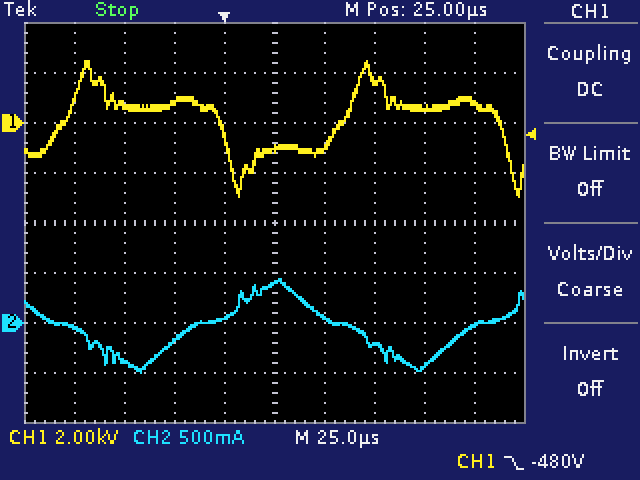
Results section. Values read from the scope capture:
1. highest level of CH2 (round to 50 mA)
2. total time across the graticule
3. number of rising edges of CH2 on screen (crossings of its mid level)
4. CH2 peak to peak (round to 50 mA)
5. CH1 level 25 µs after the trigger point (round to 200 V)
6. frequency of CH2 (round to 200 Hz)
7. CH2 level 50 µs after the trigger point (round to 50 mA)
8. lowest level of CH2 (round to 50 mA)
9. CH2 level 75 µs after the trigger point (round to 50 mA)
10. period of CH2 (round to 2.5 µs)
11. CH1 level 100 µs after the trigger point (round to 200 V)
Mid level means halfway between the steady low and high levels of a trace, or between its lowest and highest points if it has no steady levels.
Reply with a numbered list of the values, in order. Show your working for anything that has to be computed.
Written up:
1. 450 mA
2. 250 µs
3. 2
4. 450 mA − (-500 mA) = 950 mA
5. -1.0 kV
6. 1 / 140.0 µs ≈ 7.14 kHz, so 7.2 kHz to the nearest 200 Hz
7. 50 mA
8. -500 mA
9. -200 mA
10. 140.0 µs
11. 600 V
